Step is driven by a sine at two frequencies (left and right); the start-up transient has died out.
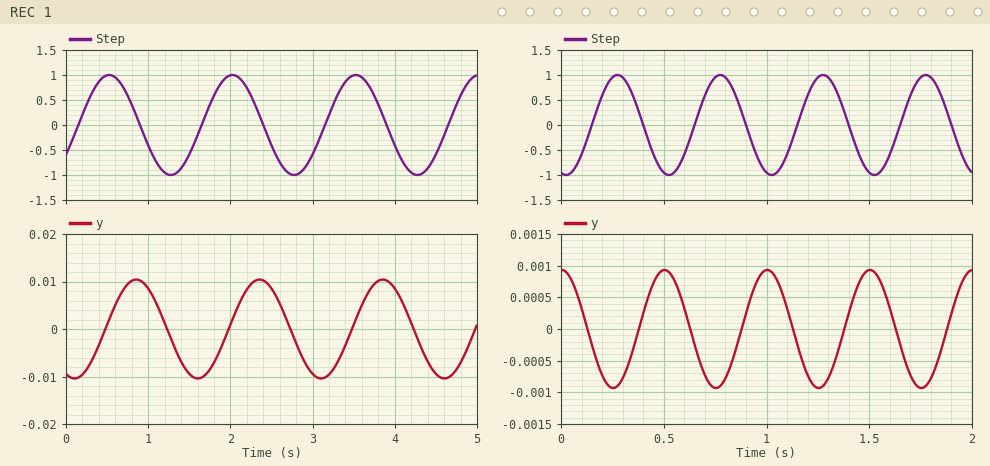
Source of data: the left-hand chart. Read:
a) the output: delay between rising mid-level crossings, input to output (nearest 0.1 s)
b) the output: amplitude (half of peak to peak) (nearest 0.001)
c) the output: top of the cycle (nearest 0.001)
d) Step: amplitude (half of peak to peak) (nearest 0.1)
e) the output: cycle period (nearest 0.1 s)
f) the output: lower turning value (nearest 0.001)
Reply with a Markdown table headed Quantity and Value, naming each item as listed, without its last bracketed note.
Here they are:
| Quantity | Value |
|---|---|
| the output: delay between rising mid-level crossings, input to output | 0.3 s |
| the output: amplitude (half of peak to peak) | 0.010 |
| the output: top of the cycle | 0.010 |
| Step: amplitude (half of peak to peak) | 1.0 |
| the output: cycle period | 1.5 s |
| the output: lower turning value | -0.010 |
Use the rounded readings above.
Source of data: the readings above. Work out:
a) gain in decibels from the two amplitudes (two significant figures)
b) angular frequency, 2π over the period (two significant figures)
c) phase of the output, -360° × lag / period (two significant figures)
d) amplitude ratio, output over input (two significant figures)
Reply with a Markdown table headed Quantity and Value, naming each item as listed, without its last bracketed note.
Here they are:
| Quantity | Value |
|---|---|
| gain in decibels from the two amplitudes | -40 dB |
| angular frequency, 2π over the period | 4.2 rad/s |
| phase of the output, -360° × lag / period | -72° |
| amplitude ratio, output over input | 0.010 |
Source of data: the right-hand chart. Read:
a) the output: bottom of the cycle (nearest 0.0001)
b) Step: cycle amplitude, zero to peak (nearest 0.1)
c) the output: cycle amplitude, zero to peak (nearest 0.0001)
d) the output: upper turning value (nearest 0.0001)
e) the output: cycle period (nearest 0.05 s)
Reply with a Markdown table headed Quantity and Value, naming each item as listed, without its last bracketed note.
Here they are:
| Quantity | Value |
|---|---|
| the output: bottom of the cycle | -0.0009 |
| Step: cycle amplitude, zero to peak | 1.0 |
| the output: cycle amplitude, zero to peak | 0.0009 |
| the output: upper turning value | 0.0009 |
| the output: cycle period | 0.50 s |
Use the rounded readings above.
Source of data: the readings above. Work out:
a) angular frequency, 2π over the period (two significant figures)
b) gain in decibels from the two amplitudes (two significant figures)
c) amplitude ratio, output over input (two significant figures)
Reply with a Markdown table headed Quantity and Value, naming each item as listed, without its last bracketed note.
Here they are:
| Quantity | Value |
|---|---|
| angular frequency, 2π over the period | 13 rad/s |
| gain in decibels from the two amplitudes | -61 dB |
| amplitude ratio, output over input | 0.00090 |
